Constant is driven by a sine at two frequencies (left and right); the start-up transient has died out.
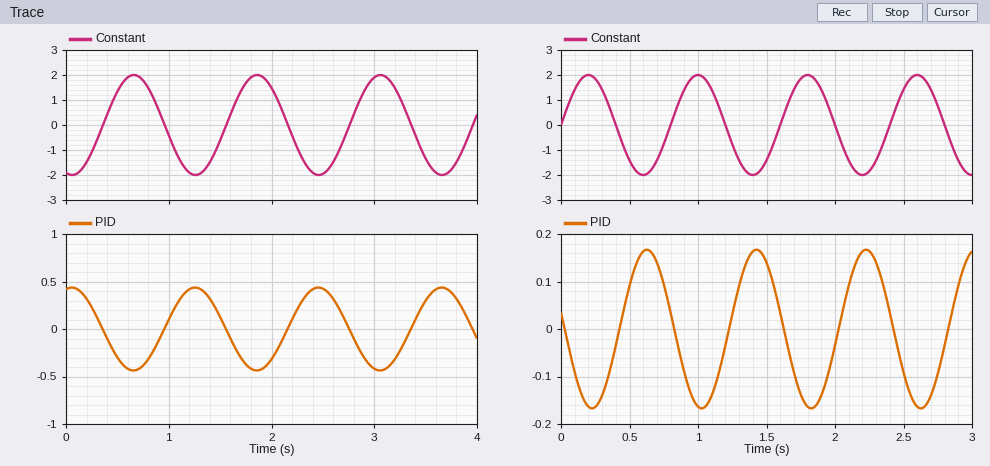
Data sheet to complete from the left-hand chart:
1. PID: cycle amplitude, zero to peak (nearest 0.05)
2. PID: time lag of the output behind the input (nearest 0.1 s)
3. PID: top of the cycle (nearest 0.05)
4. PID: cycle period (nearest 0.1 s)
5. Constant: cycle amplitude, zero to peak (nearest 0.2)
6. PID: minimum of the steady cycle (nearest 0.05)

0.45
0.6 s
0.45
1.2 s
2.0
-0.45
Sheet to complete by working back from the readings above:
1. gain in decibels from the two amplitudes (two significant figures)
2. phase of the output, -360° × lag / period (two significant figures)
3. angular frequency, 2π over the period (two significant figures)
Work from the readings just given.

-13 dB
-180°
5.2 rad/s
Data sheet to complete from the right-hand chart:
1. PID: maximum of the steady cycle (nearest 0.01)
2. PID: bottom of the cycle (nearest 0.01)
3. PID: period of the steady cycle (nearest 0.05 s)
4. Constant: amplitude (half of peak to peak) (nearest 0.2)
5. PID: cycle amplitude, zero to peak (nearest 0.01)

0.17
-0.17
0.80 s
2.0
0.17
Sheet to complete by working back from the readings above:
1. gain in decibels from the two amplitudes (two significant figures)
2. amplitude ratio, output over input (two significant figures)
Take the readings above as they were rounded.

-21 dB
0.085
